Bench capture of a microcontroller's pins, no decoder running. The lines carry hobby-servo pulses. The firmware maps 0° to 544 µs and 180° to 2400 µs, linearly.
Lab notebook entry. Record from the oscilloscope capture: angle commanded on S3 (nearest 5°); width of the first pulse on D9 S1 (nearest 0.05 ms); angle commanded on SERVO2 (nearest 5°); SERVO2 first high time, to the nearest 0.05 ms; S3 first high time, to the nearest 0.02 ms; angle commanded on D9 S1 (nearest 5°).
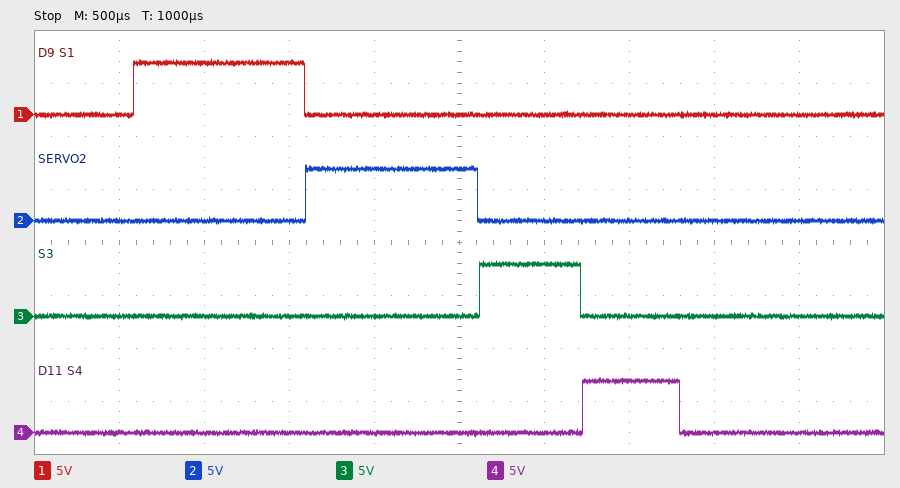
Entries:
5°
1.00 ms
45°
1.00 ms
0.60 ms
45°
